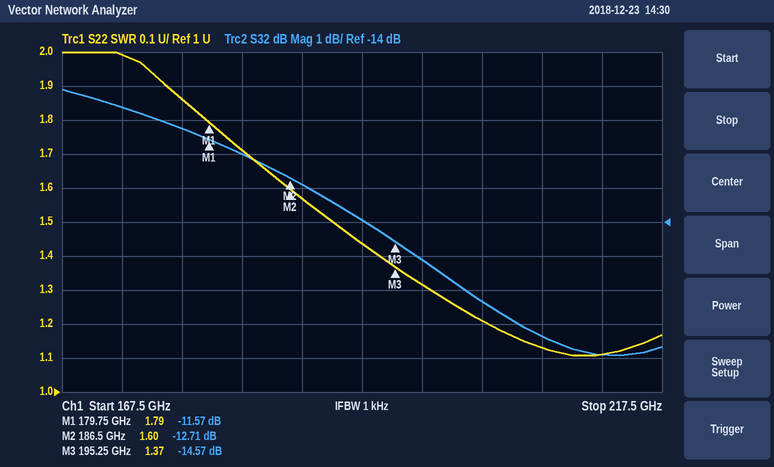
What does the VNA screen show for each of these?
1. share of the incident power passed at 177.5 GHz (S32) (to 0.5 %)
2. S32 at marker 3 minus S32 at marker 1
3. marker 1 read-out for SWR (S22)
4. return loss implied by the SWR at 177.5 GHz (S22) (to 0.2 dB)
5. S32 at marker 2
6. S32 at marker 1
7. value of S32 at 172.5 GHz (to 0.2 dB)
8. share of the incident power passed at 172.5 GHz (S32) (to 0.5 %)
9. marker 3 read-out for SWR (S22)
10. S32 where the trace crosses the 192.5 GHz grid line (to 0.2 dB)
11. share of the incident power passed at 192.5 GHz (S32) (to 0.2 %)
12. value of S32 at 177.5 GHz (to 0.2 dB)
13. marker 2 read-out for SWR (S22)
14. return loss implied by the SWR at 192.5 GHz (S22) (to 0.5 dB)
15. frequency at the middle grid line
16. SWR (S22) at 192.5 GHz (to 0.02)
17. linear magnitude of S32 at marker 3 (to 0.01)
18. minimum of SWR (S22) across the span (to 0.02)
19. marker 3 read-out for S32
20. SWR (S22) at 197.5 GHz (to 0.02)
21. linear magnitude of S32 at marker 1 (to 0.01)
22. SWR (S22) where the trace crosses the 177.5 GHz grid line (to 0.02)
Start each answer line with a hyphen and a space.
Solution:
- 7.5 %
- -3.00 dB
- 1.79
- 10.4 dB
- -12.71 dB
- -11.57 dB
- -10.6 dB
- 8.5 %
- 1.37
- -14.0 dB
- 4.0 %
- -11.2 dB
- 1.60
- 15.0 dB
- 192.5 GHz
- 1.44
- 0.19
- 1.10
- -14.57 dB
- 1.32
- 0.26
- 1.86
